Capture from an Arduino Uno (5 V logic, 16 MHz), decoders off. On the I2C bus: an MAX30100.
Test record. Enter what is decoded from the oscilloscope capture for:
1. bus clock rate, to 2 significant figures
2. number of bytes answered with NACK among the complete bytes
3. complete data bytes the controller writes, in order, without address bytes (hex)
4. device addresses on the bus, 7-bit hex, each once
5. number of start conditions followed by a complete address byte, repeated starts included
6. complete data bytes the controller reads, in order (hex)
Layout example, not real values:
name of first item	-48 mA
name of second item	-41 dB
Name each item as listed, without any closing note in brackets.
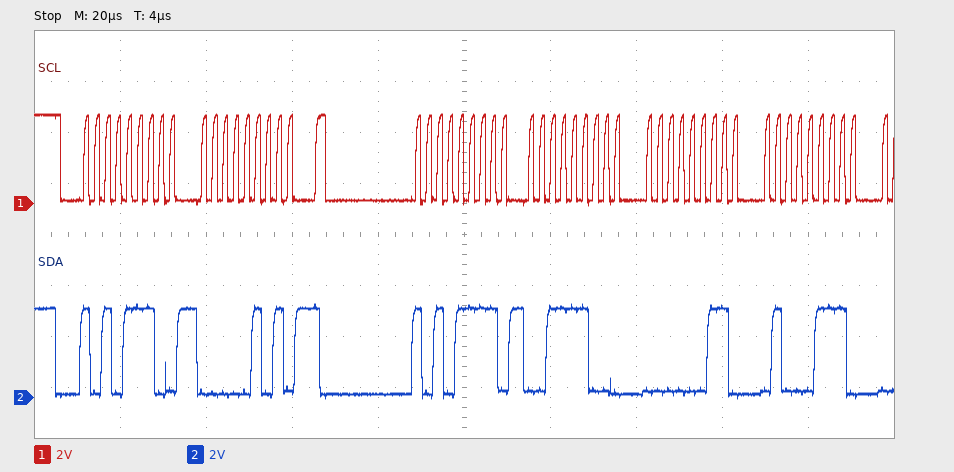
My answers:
bus clock rate, to 2 significant figures	400 kHz
number of bytes answered with NACK among the complete bytes	0
complete data bytes the controller writes, in order, without address bytes	05
device addresses on the bus, 7-bit hex, each once	0x57
number of start conditions followed by a complete address byte, repeated starts included	2
complete data bytes the controller reads, in order	3C 03 47
